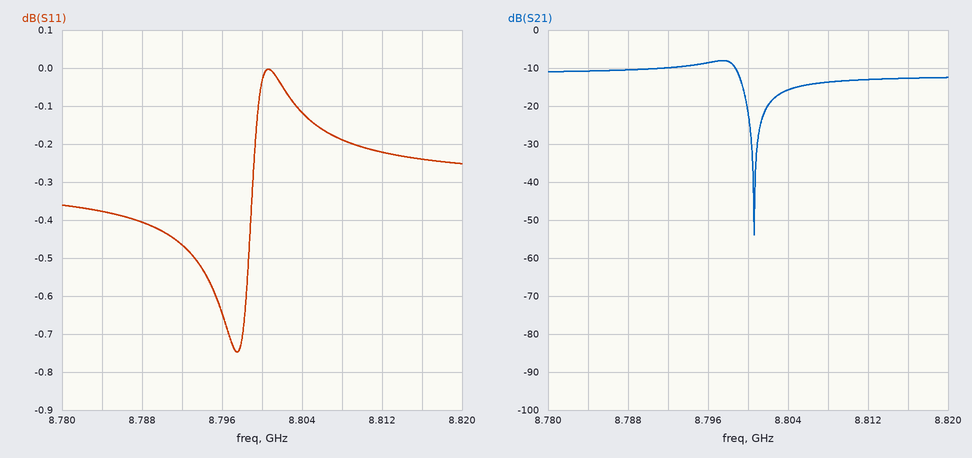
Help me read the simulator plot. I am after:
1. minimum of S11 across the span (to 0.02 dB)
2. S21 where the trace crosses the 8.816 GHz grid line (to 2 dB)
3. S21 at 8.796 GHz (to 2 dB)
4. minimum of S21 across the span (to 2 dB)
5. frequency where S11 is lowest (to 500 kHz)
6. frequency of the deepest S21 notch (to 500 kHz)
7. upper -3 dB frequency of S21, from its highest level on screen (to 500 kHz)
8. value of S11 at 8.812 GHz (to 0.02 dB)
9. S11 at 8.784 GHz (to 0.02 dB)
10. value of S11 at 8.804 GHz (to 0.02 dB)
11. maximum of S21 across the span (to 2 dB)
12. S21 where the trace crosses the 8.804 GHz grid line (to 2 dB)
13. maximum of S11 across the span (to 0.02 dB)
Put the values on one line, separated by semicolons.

-0.74 dB; -12 dB; -8 dB; -54 dB; 8.7975 GHz; 8.8005 GHz; 8.7990 GHz; -0.22 dB; -0.38 dB; -0.12 dB; -8 dB; -16 dB; 0.00 dB
